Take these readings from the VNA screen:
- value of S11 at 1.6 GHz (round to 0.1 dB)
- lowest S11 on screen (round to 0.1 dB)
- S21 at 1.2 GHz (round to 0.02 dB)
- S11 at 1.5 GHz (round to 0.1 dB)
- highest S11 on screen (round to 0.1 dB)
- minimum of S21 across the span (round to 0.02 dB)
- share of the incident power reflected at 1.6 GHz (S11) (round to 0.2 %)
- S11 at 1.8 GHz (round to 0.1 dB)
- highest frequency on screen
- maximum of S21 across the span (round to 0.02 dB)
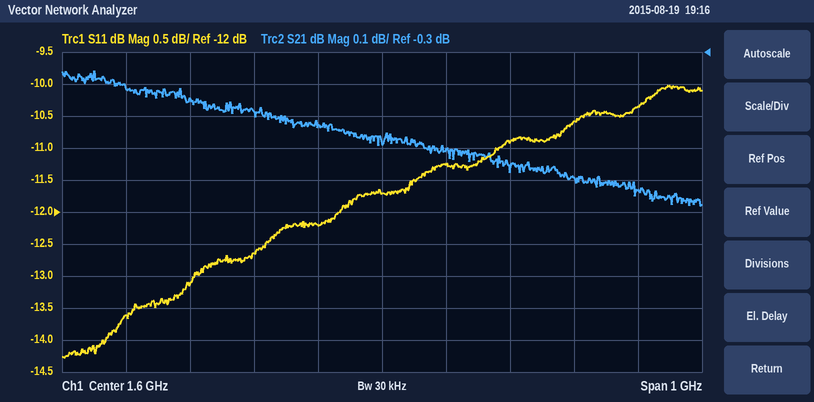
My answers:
-11.7 dB
-14.3 dB
-0.42 dB
-12.2 dB
-10.0 dB
-0.78 dB
6.8 %
-10.9 dB
2.1 GHz
-0.36 dB
